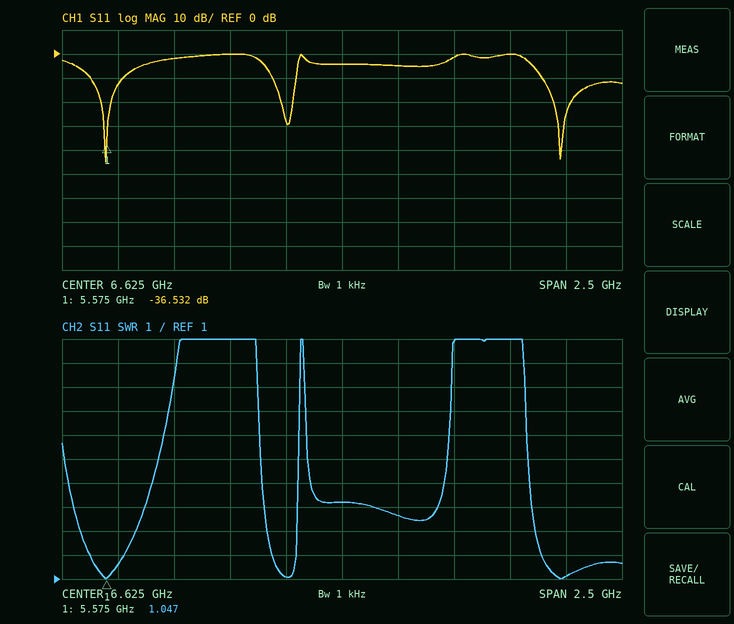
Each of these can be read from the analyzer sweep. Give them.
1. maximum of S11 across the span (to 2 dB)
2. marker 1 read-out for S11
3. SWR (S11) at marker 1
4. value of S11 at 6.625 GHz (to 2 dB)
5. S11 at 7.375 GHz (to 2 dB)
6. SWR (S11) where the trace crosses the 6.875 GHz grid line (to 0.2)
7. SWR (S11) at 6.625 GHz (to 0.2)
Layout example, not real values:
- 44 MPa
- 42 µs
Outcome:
- 0 dB
- -36.532 dB
- 1.047
- -4 dB
- 0 dB
- 3.6
- 4.2
